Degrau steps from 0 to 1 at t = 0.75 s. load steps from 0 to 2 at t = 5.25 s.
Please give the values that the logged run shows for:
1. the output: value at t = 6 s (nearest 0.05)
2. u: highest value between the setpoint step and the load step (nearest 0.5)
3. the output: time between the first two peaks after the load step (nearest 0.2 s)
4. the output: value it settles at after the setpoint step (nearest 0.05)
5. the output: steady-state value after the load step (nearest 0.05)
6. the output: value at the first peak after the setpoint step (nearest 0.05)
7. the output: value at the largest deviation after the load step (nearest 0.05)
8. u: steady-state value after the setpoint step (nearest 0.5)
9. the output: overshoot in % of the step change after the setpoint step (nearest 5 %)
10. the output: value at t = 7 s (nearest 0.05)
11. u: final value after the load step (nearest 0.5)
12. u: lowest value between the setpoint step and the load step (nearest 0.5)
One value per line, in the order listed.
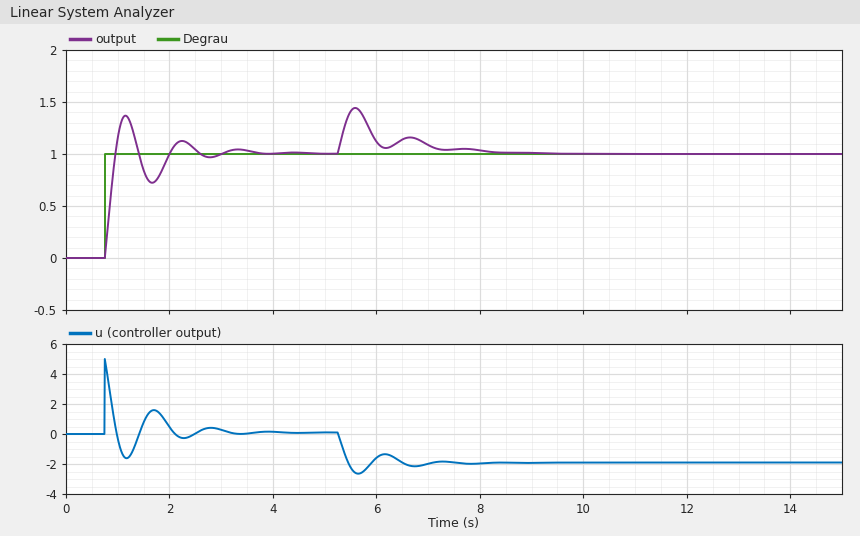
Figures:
1.10
5.0
1.0 s
1.00
1.00
1.35
1.45
0.0
35 %
1.10
-2.0
-1.5
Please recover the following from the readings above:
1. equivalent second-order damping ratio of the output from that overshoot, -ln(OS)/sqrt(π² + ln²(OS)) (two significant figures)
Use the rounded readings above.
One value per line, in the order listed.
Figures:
0.32
